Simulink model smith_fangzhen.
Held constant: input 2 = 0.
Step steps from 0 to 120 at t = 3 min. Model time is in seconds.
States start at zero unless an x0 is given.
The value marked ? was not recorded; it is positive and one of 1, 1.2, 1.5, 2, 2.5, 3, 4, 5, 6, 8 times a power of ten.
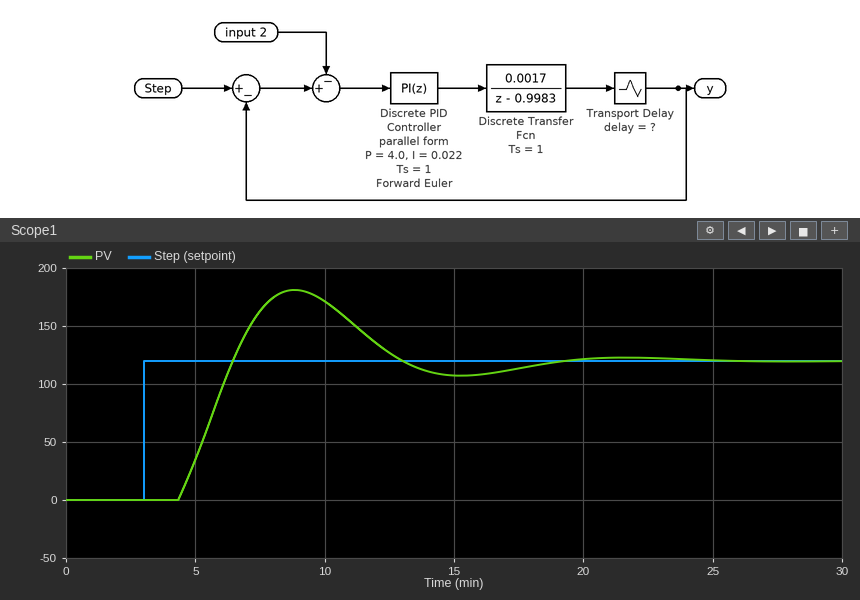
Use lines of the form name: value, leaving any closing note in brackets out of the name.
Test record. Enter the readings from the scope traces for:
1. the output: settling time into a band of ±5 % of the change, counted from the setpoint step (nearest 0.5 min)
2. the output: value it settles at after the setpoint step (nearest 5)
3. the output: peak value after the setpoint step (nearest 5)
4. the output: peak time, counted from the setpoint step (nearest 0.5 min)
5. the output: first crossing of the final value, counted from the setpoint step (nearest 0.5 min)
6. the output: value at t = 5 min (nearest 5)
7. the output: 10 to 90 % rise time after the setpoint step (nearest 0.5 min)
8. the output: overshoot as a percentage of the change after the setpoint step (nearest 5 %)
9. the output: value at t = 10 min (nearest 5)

the output: settling time into a band of ±5 % of the change, counted from the setpoint step: 14.5 min
the output: value it settles at after the setpoint step: 120
the output: peak value after the setpoint step: 180
the output: peak time, counted from the setpoint step: 6.0 min
the output: first crossing of the final value, counted from the setpoint step: 3.5 min
the output: value at t = 5 min: 35
the output: 10 to 90 % rise time after the setpoint step: 1.5 min
the output: overshoot as a percentage of the change after the setpoint step: 50 %
the output: value at t = 10 min: 170
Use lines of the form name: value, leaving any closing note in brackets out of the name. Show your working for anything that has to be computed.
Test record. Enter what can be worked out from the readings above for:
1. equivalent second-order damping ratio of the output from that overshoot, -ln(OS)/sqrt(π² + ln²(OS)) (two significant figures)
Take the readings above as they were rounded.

equivalent second-order damping ratio of the output from that overshoot, -ln(OS)/sqrt(π² + ln²(OS)): ln(0.5) = -0.693; 0.693 / sqrt(9.870 + 0.480) = 0.22
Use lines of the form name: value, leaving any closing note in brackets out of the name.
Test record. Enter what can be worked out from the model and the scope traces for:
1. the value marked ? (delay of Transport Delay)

the value marked ?: 80
